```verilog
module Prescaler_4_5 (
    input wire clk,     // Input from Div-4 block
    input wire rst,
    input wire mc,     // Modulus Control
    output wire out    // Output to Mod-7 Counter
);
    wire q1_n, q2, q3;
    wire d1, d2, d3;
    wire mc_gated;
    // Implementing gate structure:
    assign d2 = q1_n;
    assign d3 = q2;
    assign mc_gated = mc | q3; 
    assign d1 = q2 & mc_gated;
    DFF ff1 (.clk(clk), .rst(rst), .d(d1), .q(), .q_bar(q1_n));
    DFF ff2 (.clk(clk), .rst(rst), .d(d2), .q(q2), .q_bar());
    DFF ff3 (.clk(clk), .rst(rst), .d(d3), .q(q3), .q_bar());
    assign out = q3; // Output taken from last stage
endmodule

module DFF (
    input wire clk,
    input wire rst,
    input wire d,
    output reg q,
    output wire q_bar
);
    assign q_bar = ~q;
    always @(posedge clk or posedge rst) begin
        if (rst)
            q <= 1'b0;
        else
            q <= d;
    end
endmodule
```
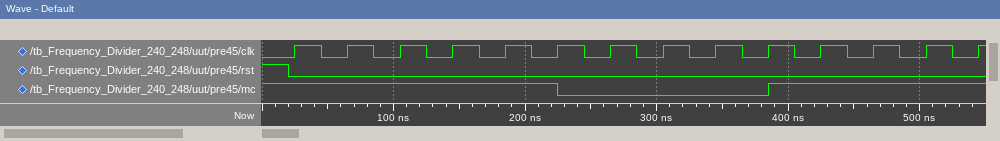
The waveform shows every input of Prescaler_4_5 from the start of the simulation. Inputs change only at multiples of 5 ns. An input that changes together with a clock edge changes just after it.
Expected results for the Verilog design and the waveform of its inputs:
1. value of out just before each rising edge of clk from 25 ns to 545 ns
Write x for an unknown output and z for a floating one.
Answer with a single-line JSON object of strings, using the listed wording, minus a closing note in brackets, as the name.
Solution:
{"value of out just before each rising edge of clk from 25 ns to 545 ns": "0 0 1 1 0 0 1 1 0 0 1 1 1 0"}
